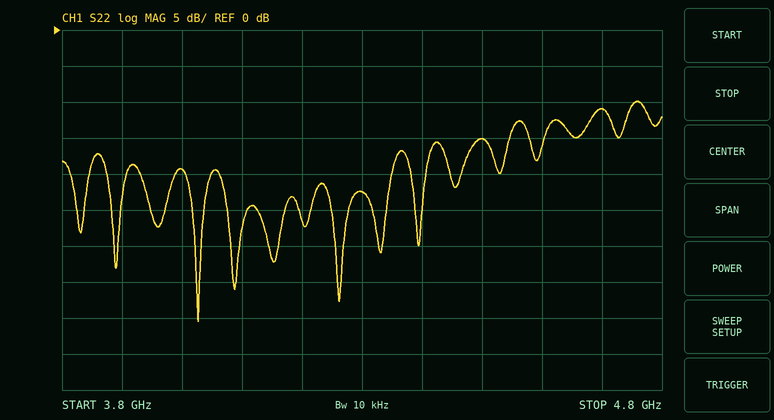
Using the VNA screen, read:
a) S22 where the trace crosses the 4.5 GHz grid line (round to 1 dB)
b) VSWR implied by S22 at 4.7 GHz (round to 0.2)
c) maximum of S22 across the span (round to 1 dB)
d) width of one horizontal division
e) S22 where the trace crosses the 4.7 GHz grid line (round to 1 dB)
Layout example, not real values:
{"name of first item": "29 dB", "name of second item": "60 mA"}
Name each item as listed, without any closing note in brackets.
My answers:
{"S22 where the trace crosses the 4.5 GHz grid line": "-15 dB", "VSWR implied by S22 at 4.7 GHz": "1.8", "maximum of S22 across the span": "-10 dB", "width of one horizontal division": "100 MHz", "S22 where the trace crosses the 4.7 GHz grid line": "-11 dB"}
